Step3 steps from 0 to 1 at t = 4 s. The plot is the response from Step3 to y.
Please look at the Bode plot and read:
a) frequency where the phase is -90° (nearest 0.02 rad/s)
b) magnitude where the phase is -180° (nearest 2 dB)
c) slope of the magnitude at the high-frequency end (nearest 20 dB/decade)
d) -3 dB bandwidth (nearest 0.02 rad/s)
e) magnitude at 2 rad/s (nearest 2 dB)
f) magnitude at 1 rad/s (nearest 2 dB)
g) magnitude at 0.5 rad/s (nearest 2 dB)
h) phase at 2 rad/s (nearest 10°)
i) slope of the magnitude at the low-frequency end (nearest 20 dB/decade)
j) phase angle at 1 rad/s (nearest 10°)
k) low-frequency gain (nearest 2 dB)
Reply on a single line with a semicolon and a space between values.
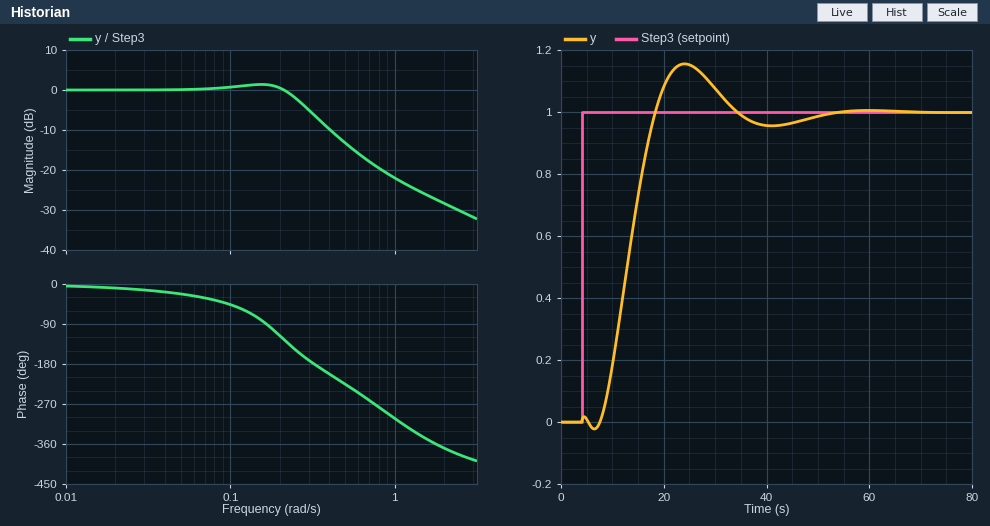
0.16 rad/s; -6 dB; -20 dB/decade; 0.26 rad/s; -28 dB; -22 dB; -14 dB; -370°; 0 dB/decade; -300°; 0 dB
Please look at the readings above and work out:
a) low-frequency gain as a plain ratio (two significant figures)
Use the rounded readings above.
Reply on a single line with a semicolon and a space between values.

1.0
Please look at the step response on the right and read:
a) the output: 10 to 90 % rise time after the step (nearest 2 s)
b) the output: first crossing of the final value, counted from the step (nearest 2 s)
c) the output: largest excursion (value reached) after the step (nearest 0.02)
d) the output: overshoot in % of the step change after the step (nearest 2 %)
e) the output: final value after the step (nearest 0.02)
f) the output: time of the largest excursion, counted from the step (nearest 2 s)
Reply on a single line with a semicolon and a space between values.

8 s; 14 s; 1.16; 16 %; 1.00; 20 s
